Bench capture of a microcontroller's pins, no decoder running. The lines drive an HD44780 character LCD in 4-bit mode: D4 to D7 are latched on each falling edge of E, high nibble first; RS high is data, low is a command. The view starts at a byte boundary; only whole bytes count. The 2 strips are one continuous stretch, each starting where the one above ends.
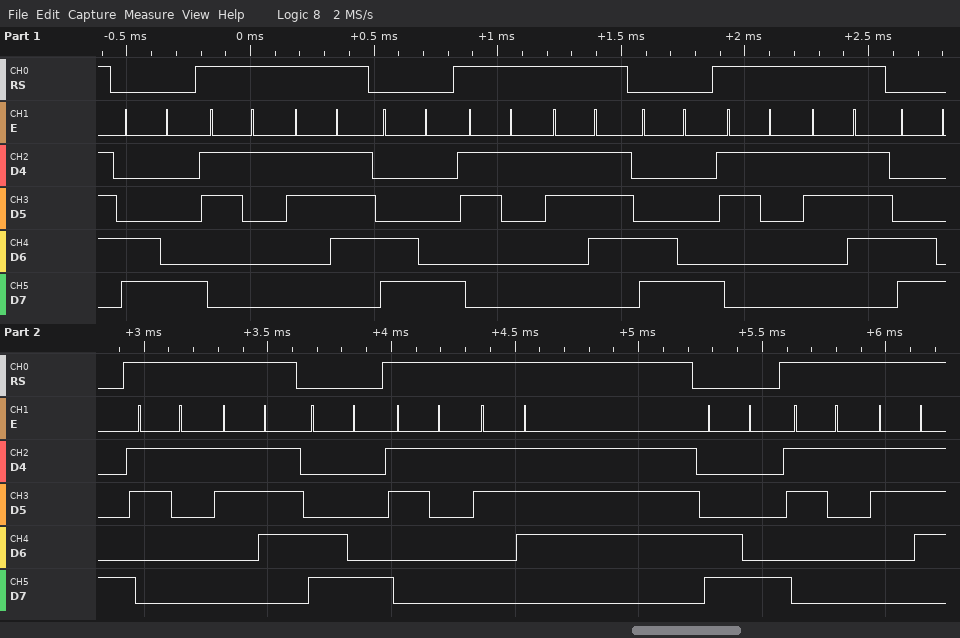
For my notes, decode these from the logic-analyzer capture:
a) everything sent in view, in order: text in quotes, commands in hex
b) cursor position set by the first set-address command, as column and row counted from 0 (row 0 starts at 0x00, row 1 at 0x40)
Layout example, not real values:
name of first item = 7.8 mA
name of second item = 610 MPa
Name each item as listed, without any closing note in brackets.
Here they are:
everything sent in view, in order: text in quotes, commands in hex = 0xC8 "17" 0xC8 "17" 0xC8 "17" 0xC8 "17" 0xC8 "17" 0xC8 "17"
cursor position set by the first set-address command, as column and row counted from 0 = column 8, row 1
